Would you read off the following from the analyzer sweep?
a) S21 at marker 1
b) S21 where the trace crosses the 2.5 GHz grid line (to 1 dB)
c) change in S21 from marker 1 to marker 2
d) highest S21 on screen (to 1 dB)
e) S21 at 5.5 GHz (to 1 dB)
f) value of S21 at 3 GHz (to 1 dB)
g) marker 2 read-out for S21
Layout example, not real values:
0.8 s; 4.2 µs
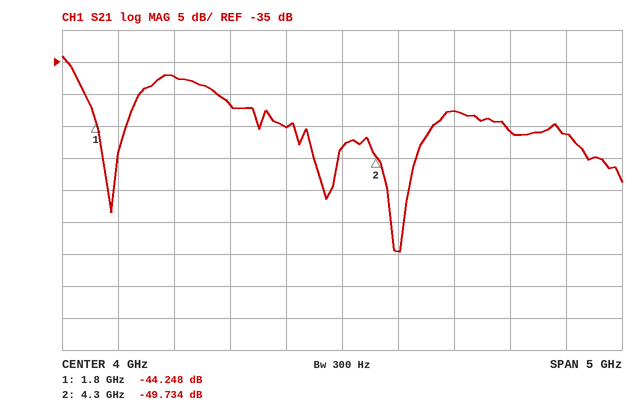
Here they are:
-44.248 dB; -37 dB; -5.486 dB; -34 dB; -46 dB; -42 dB; -49.734 dB
